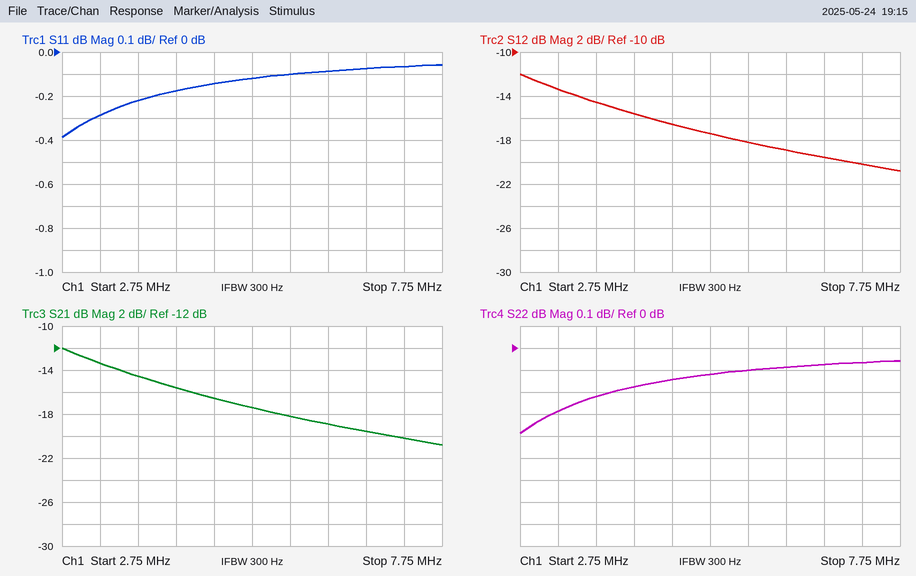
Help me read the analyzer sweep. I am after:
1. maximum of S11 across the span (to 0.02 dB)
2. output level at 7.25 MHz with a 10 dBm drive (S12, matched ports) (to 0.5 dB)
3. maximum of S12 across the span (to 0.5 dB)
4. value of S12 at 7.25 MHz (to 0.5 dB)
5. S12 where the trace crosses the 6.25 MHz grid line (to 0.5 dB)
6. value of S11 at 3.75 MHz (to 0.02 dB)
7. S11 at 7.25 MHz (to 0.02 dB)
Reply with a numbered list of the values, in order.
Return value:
1. -0.06 dB
2. -10.0 dBm
3. -12.0 dB
4. -20.0 dB
5. -19.0 dB
6. -0.22 dB
7. -0.06 dB
